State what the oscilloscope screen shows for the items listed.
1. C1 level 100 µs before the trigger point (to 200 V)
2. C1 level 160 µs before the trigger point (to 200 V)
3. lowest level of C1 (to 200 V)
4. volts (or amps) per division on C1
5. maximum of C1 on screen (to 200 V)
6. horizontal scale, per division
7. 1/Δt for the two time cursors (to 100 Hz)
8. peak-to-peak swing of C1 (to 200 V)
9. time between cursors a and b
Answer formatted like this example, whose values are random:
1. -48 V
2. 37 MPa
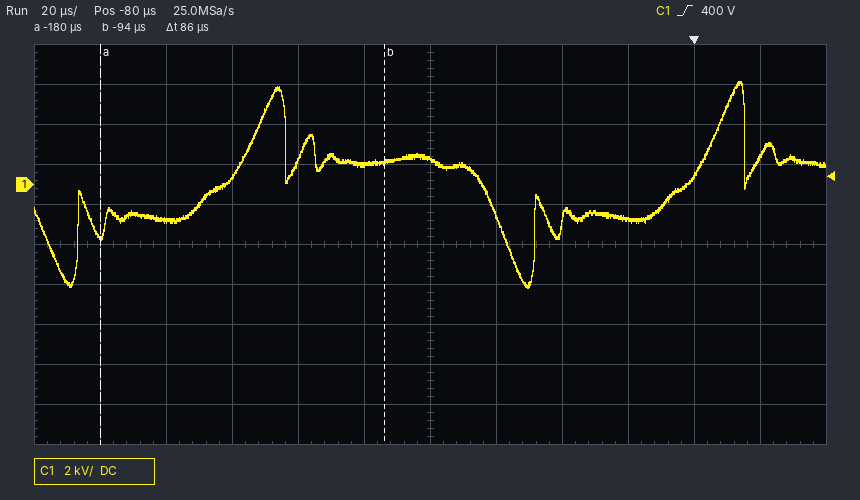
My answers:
1. 1.0 kV
2. -1.8 kV
3. -5.2 kV
4. 2 kV
5. 5.2 kV
6. 20 µs
7. 11.6 kHz
8. 10.4 kV
9. 86 µs
